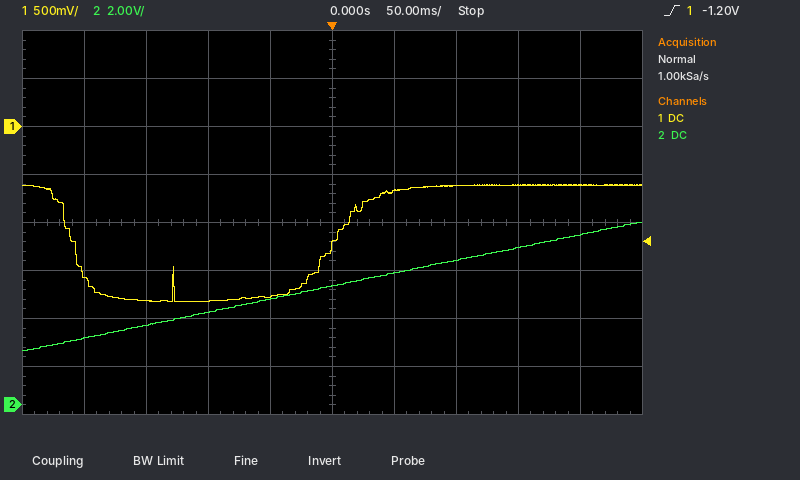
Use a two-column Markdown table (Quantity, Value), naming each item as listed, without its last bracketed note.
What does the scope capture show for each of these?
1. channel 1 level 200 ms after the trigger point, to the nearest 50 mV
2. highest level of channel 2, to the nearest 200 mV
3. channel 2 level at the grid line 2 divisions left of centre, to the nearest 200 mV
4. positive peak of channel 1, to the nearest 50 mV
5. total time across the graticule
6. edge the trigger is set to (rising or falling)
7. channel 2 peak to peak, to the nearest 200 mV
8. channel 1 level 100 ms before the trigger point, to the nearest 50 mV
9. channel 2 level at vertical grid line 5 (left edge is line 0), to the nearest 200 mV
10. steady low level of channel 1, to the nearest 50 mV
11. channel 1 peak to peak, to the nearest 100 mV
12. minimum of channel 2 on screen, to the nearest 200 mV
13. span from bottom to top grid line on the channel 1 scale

| Quantity | Value |
|---|---|
| channel 1 level 200 ms after the trigger point, to the nearest 50 mV | -600 mV |
| highest level of channel 2, to the nearest 200 mV | 7.6 V |
| channel 2 level at the grid line 2 divisions left of centre, to the nearest 200 mV | 3.8 V |
| positive peak of channel 1, to the nearest 50 mV | -600 mV |
| total time across the graticule | 500 ms |
| edge the trigger is set to | rising |
| channel 2 peak to peak, to the nearest 200 mV | 5.4 V |
| channel 1 level 100 ms before the trigger point, to the nearest 50 mV | -1.80 V |
| channel 2 level at vertical grid line 5 (left edge is line 0), to the nearest 200 mV | 5.0 V |
| steady low level of channel 1, to the nearest 50 mV | -1.80 V |
| channel 1 peak to peak, to the nearest 100 mV | 1.20 V |
| minimum of channel 2 on screen, to the nearest 200 mV | 2.2 V |
| span from bottom to top grid line on the channel 1 scale | 4 V |
